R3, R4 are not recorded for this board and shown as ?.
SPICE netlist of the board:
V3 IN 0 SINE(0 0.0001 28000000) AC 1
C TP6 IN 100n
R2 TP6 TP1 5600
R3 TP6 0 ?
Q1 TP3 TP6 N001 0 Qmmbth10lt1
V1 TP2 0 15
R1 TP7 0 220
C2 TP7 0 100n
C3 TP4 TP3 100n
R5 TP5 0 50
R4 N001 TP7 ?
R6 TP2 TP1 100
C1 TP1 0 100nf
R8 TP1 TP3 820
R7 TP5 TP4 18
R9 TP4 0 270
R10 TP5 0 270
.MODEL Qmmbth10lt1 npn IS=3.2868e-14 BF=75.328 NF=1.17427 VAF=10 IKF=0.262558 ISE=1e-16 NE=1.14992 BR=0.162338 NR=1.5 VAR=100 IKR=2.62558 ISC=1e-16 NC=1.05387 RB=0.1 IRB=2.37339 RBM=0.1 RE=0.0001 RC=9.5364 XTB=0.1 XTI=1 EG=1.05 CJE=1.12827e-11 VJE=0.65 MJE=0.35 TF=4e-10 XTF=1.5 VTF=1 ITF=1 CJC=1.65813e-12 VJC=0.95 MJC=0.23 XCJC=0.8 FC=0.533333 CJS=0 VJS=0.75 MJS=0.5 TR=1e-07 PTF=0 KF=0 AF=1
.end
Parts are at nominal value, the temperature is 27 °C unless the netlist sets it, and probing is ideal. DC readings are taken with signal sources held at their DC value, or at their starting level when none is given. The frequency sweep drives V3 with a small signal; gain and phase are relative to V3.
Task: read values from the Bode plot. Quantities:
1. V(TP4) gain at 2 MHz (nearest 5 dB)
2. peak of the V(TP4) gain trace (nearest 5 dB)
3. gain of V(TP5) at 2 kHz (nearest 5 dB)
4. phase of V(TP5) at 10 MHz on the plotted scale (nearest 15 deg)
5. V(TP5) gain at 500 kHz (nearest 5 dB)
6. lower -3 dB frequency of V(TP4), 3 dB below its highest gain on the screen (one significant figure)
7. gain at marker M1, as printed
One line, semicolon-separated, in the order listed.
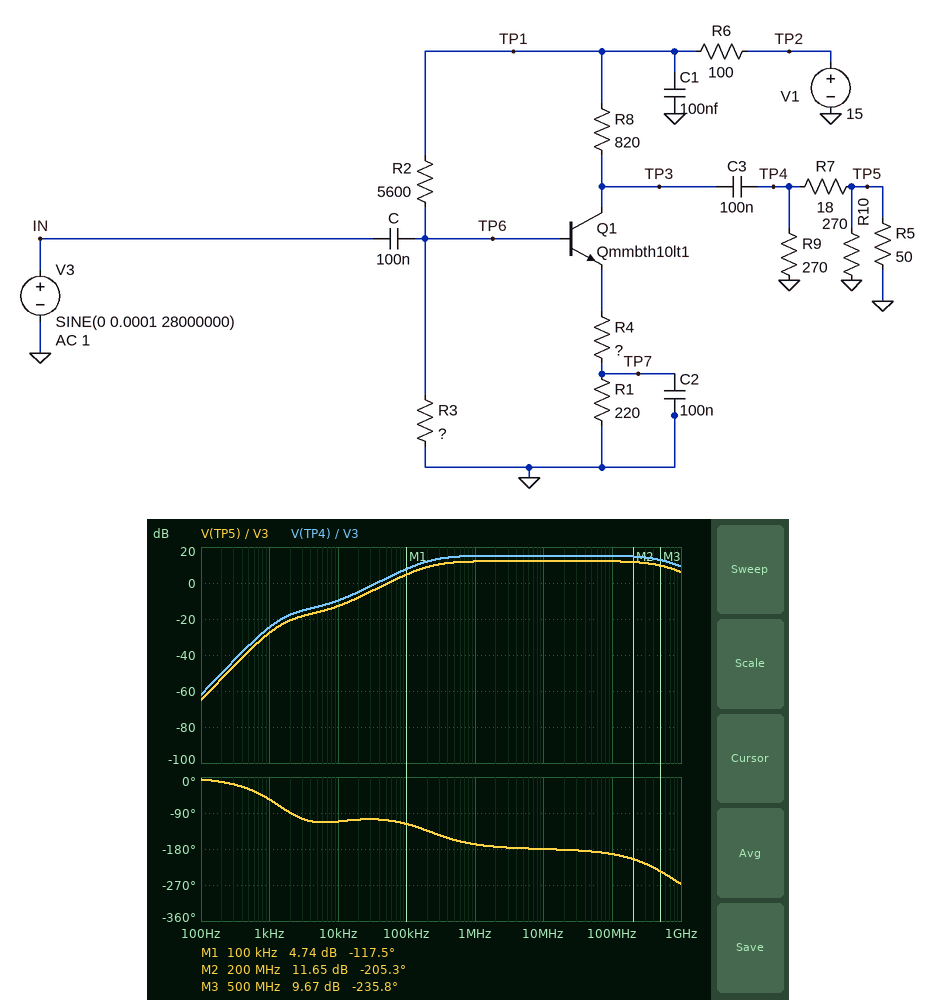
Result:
15 dB; 15 dB; -20 dB; -180 deg; 10 dB; 200 kHz; 4.74 dB
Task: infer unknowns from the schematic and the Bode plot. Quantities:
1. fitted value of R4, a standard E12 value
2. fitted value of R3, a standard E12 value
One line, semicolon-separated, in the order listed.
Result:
4.7 Ω; 1.8 kΩ
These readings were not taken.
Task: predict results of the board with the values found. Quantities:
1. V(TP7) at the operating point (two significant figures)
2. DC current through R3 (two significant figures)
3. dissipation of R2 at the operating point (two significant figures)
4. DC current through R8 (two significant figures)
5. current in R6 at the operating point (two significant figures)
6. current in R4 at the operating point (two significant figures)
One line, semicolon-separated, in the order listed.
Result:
2.3 V; 1.7 mA; 20 mW; 10 mA; 12 mA; 10 mA
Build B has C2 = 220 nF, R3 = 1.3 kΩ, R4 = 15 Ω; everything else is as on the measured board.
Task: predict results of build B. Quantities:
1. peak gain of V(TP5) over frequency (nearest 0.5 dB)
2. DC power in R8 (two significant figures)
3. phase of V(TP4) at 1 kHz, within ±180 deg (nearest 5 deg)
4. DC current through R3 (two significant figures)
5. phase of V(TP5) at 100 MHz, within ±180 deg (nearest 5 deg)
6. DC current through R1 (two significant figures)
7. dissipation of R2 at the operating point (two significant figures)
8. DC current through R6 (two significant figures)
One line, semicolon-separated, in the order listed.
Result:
4.5 dB; 45 mW; -45 deg; 2.0 mA; 165 deg; 7.5 mA; 24 mW; 9.5 mA
